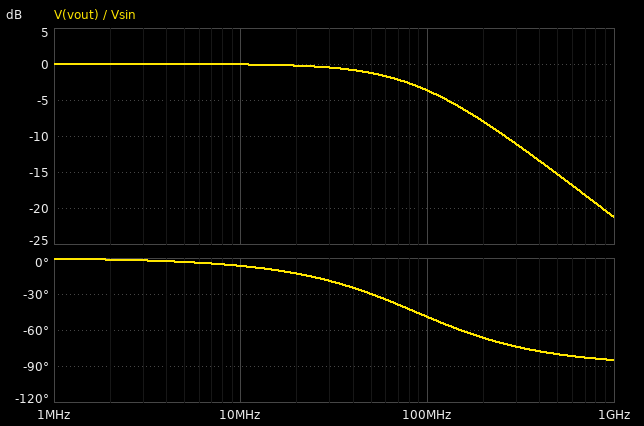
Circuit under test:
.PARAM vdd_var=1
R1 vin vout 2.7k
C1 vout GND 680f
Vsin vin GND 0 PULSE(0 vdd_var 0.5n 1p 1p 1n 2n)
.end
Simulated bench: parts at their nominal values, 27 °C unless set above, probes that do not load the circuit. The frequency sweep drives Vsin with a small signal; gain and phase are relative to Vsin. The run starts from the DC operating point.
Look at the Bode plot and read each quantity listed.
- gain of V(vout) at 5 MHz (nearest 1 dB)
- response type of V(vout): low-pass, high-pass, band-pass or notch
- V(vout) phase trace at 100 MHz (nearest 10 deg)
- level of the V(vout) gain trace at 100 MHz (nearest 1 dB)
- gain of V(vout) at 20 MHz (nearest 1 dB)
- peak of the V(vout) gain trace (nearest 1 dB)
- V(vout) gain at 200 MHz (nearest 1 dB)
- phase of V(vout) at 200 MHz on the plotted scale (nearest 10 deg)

0 dB
low-pass
-50 deg
-4 dB
0 dB
0 dB
-8 dB
-70 deg
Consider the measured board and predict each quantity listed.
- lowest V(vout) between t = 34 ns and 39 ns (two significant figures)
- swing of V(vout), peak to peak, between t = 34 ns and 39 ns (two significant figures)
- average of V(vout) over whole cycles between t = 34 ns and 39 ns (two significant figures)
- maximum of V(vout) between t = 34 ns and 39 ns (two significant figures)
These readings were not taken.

370 mV
270 mV
500 mV
630 mV
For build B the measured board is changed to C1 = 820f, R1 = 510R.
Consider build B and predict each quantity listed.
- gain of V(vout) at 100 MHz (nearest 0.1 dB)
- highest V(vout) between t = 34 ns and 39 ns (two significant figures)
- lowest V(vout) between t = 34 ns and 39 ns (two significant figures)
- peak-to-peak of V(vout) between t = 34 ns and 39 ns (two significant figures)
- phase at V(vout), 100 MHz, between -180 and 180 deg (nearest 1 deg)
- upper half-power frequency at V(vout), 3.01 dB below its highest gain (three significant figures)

-0.3 dB
920 mV
84 mV
830 mV
-15 deg
381 MHz
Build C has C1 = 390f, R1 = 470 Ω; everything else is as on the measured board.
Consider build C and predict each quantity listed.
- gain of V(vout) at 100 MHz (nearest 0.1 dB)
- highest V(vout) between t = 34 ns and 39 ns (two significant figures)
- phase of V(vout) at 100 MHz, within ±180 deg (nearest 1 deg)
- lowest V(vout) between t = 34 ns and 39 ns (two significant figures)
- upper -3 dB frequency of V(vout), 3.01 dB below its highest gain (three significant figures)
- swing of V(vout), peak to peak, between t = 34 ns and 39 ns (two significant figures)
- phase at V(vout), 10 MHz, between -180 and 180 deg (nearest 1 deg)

-0.1 dB
1.0 V
-7 deg
4.3 mV
868 MHz
990 mV
-1 deg
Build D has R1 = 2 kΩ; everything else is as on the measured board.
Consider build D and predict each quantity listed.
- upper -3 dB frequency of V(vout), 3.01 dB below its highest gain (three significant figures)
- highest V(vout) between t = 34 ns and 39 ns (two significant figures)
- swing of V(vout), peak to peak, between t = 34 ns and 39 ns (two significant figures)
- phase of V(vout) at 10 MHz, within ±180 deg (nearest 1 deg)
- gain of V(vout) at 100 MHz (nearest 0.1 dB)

117 MHz
680 mV
350 mV
-5 deg
-2.4 dB
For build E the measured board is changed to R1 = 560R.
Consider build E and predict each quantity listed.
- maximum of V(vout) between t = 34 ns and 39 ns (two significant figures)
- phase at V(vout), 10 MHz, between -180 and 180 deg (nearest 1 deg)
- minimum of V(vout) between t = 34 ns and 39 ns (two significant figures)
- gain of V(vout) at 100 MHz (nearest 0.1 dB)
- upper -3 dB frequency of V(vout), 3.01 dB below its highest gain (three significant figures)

930 mV
-1 deg
68 mV
-0.2 dB
418 MHz
